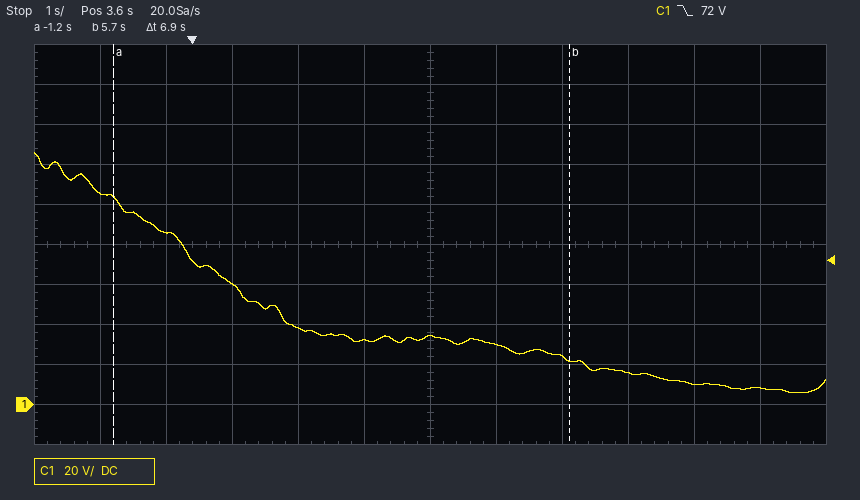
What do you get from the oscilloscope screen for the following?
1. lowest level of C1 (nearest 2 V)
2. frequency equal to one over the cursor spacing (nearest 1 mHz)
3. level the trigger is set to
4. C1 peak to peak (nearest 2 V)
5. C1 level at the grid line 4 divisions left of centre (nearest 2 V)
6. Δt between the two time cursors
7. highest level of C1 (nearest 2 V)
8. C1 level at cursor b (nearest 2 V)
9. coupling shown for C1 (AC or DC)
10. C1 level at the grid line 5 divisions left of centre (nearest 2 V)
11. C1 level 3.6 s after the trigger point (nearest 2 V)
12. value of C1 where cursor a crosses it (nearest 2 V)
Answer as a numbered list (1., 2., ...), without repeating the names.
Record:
1. 6 V
2. 145 mHz
3. 72 V
4. 120 V
5. 86 V
6. 6.9 s
7. 126 V
8. 22 V
9. DC
10. 106 V
11. 34 V
12. 104 V
